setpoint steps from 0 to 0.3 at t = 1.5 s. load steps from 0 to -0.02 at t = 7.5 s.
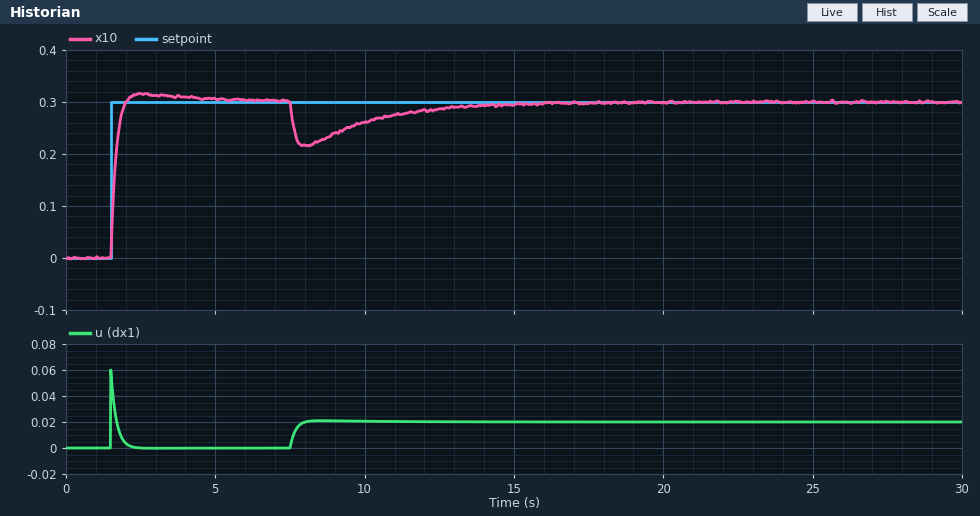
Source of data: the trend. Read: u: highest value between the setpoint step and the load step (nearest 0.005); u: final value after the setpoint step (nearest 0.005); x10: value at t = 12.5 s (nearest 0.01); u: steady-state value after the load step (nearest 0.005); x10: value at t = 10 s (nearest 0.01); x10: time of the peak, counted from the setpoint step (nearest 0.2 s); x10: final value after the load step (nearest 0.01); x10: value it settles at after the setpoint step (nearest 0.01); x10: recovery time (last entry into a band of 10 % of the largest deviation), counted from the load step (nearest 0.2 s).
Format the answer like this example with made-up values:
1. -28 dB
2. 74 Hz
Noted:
1. 0.060
2. 0.000
3. 0.29
4. 0.020
5. 0.26
6. 1.0 s
7. 0.30
8. 0.30
9. 6.0 s
